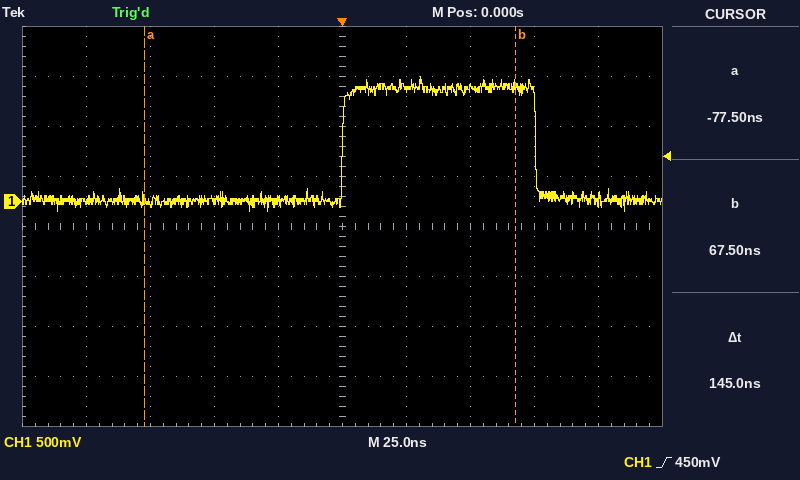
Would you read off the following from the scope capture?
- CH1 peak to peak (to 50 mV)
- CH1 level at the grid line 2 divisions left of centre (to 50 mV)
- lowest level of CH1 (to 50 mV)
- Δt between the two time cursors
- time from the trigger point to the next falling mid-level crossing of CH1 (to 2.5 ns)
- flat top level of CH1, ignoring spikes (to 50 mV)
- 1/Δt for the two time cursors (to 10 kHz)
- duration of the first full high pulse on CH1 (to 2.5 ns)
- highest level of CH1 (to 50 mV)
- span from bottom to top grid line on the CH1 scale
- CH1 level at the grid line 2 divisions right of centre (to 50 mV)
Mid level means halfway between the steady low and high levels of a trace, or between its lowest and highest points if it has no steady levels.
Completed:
1.35 V
0 mV
-100 mV
145 ns
75.0 ns
1.15 V
6.90 MHz
75.0 ns
1.25 V
4 V
1.15 V
